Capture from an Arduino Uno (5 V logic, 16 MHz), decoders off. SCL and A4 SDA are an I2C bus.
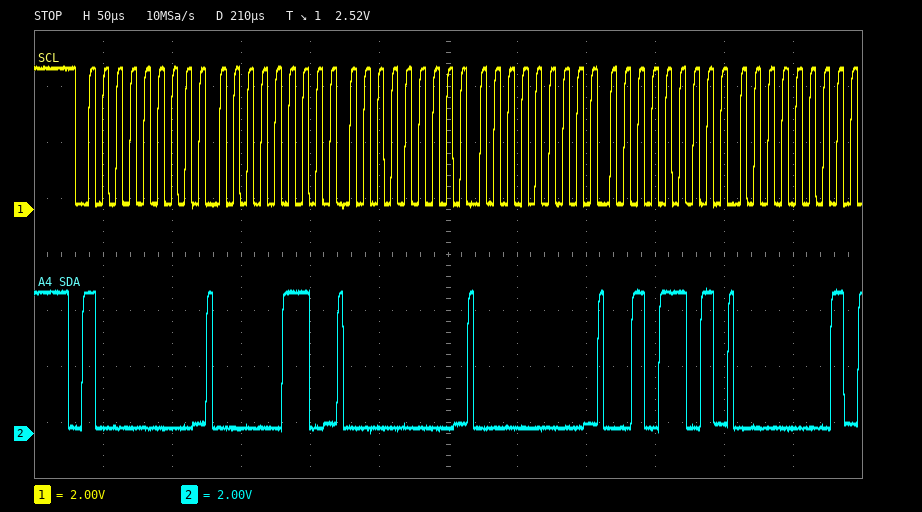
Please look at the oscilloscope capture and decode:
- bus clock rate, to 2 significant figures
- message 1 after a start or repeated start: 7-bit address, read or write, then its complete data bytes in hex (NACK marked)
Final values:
100 kHz
0x40 write: 06 00 00 2D 01
